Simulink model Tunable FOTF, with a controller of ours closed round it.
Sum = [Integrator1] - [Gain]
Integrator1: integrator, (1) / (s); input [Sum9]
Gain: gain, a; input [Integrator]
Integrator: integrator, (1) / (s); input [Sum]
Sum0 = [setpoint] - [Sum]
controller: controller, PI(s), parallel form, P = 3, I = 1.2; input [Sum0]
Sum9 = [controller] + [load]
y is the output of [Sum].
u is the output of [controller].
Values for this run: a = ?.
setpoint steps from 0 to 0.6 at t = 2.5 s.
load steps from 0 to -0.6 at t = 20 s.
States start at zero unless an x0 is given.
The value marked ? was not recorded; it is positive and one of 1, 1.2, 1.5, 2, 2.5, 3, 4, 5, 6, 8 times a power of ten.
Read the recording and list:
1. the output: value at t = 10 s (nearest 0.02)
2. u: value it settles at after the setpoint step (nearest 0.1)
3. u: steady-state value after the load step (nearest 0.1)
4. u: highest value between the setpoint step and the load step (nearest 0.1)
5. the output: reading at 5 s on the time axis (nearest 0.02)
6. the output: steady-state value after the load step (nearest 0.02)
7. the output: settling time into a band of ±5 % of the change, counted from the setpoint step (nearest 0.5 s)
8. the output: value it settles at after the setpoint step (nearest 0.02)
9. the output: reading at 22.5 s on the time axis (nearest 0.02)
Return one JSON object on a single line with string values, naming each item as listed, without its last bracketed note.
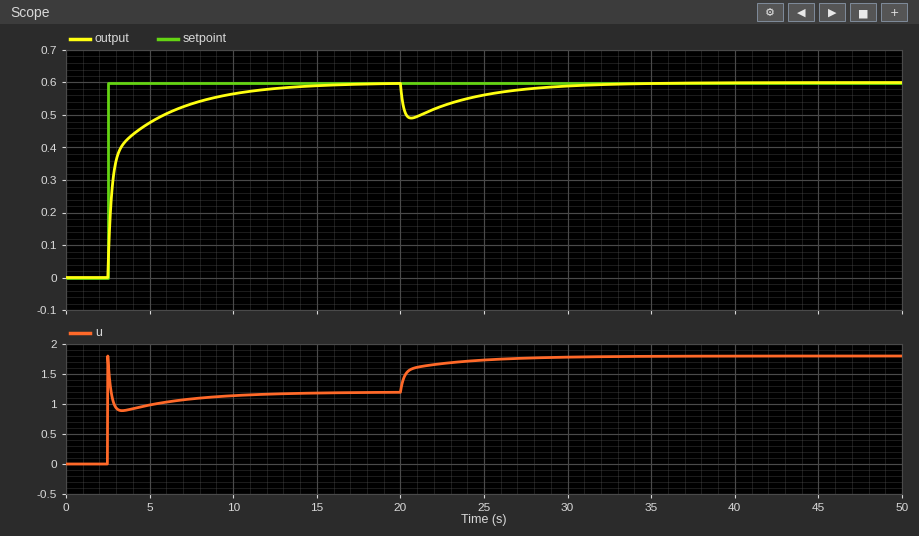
{"the output: value at t = 10 s": "0.56", "u: value it settles at after the setpoint step": "1.2", "u: steady-state value after the load step": "1.8", "u: highest value between the setpoint step and the load step": "1.8", "the output: reading at 5 s on the time axis": "0.48", "the output: steady-state value after the load step": "0.60", "the output: settling time into a band of ±5 % of the change, counted from the setpoint step": "8.0 s", "the output: value it settles at after the setpoint step": "0.60", "the output: reading at 22.5 s on the time axis": "0.52"}
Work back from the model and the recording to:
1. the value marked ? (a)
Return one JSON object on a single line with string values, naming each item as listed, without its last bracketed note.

{"the value marked ?": "2"}
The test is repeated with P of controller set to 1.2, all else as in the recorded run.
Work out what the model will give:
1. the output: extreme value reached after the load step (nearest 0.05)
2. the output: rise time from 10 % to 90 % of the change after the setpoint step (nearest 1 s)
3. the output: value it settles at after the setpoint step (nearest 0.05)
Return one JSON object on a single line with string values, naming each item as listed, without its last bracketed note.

{"the output: extreme value reached after the load step": "0.45", "the output: rise time from 10 % to 90 % of the change after the setpoint step": "4 s", "the output: value it settles at after the setpoint step": "0.60"}
